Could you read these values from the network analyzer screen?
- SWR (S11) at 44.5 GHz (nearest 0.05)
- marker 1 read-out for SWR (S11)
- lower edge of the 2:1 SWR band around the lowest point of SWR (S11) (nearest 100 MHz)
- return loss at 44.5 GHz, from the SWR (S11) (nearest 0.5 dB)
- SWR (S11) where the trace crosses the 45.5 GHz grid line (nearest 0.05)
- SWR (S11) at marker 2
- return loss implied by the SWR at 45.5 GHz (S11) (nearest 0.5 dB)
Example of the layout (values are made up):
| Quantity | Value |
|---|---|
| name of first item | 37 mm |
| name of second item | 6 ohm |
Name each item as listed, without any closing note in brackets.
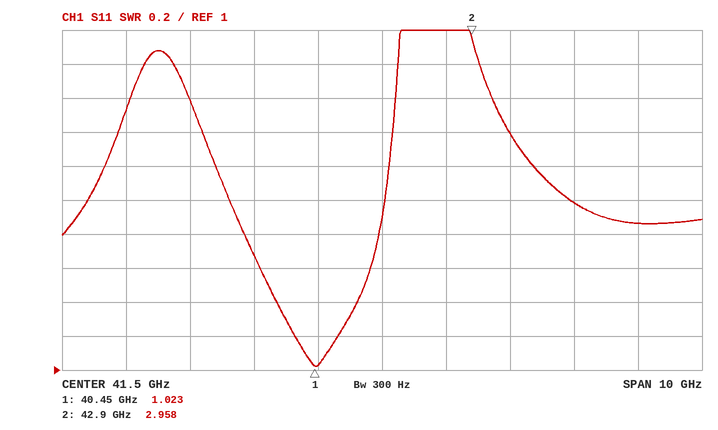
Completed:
| Quantity | Value |
|---|---|
| SWR (S11) at 44.5 GHz | 2.00 |
| marker 1 read-out for SWR | 1.023 |
| lower edge of the 2:1 SWR band around the lowest point of SWR (S11) | 39.1 GHz |
| return loss at 44.5 GHz, from the SWR (S11) | 9.5 dB |
| SWR (S11) where the trace crosses the 45.5 GHz grid line | 1.85 |
| SWR (S11) at marker 2 | 2.958 |
| return loss implied by the SWR at 45.5 GHz (S11) | 10.5 dB |
